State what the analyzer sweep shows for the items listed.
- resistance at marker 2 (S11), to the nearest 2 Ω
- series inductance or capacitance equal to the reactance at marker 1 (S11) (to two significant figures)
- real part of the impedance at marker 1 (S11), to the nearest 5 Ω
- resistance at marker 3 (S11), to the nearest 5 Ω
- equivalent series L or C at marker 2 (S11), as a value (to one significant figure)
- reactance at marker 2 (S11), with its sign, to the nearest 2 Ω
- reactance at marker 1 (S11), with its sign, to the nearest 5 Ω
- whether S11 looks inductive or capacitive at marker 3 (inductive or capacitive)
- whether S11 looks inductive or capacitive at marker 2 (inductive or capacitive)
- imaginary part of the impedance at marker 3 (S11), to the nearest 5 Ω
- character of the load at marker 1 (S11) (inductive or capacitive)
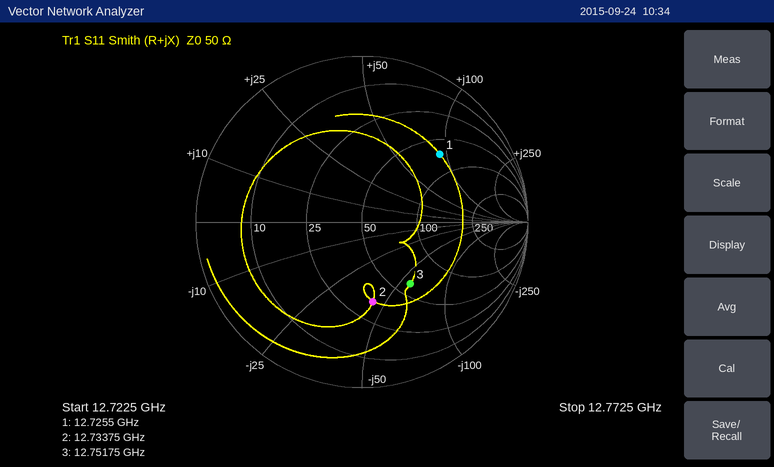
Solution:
34 Ω
1.1 nH
70 Ω
60 Ω
300 fF
-44 Ω
+90 Ω
capacitive
capacitive
-60 Ω
inductive
